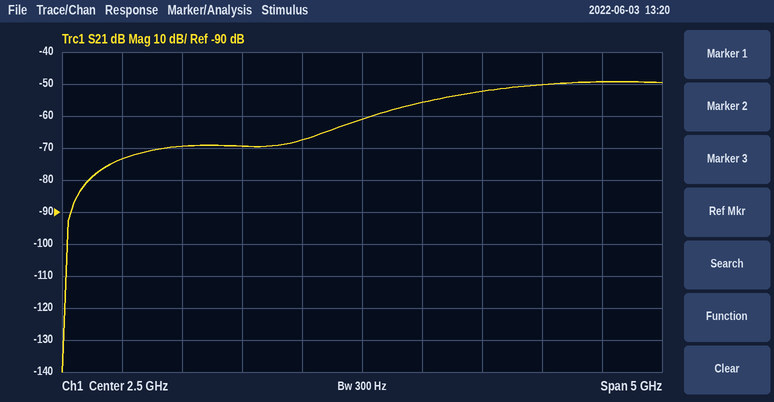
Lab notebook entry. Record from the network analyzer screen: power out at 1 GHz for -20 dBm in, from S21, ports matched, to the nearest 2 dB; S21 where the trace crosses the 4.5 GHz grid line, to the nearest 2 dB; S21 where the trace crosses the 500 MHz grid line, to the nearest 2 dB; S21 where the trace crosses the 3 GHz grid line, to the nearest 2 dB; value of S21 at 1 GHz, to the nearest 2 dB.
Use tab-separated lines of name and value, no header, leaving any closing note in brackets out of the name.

power out at 1 GHz for -20 dBm in, from S21, ports matched, to the nearest 2 dB	-90 dBm
S21 where the trace crosses the 4.5 GHz grid line, to the nearest 2 dB	-50 dB
S21 where the trace crosses the 500 MHz grid line, to the nearest 2 dB	-74 dB
S21 where the trace crosses the 3 GHz grid line, to the nearest 2 dB	-56 dB
value of S21 at 1 GHz, to the nearest 2 dB	-70 dB
